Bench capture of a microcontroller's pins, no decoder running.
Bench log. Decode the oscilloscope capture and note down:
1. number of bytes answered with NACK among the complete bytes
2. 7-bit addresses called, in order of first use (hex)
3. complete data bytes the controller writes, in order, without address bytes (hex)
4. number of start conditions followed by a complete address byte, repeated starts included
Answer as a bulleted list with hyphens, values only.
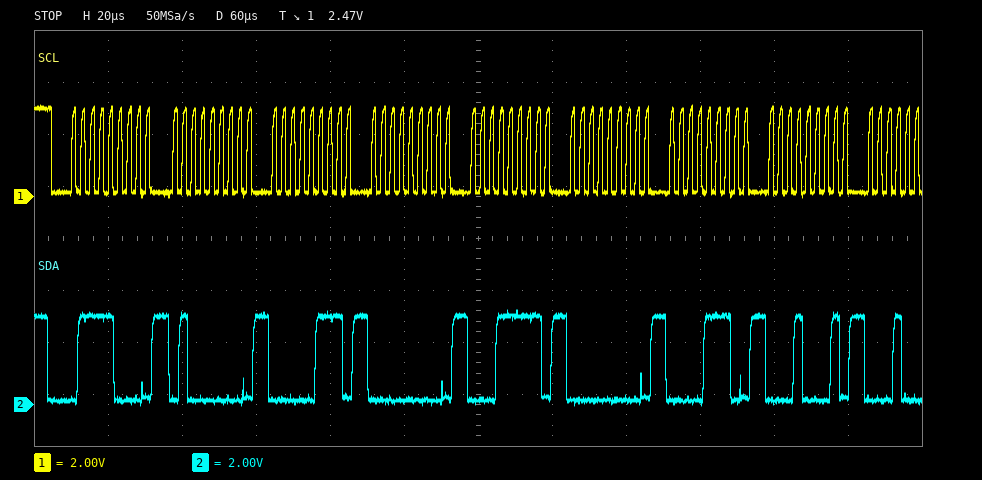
- 0
- 0x3C
- 40 07 00 1F 00 0E 11
- 1
